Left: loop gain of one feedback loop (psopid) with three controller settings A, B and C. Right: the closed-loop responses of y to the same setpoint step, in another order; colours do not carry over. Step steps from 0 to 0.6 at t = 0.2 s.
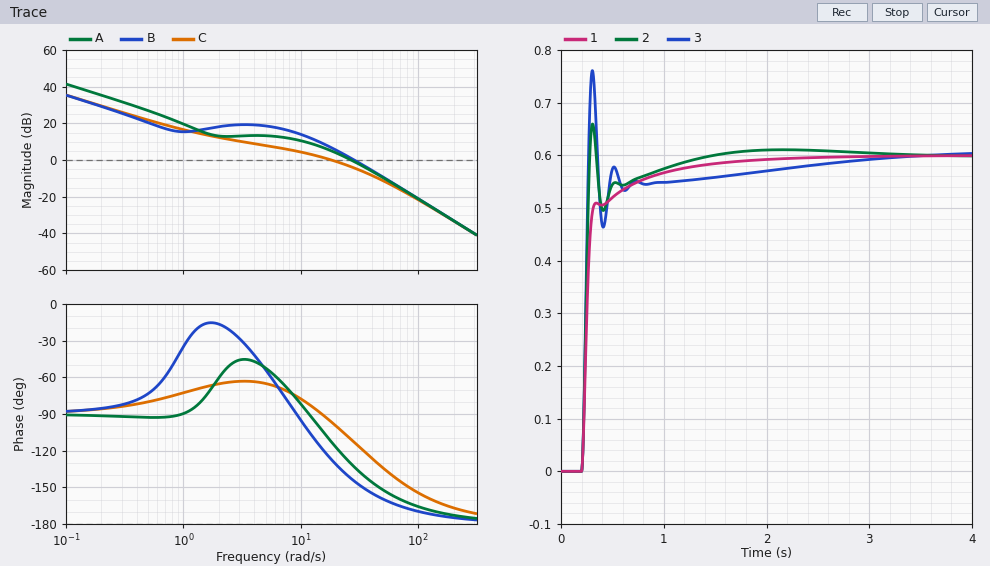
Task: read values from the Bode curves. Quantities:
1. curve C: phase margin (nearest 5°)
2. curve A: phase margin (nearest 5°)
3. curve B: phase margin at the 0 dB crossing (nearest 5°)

85°
50°
35°
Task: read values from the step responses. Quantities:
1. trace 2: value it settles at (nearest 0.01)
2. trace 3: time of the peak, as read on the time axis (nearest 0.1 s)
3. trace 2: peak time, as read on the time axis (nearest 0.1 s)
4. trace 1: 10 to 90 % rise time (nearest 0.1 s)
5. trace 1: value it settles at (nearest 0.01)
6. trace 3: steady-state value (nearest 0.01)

0.60
0.3 s
0.3 s
0.4 s
0.60
0.60
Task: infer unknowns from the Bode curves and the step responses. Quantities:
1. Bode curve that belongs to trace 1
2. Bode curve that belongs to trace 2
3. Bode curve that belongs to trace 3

C
A
B
